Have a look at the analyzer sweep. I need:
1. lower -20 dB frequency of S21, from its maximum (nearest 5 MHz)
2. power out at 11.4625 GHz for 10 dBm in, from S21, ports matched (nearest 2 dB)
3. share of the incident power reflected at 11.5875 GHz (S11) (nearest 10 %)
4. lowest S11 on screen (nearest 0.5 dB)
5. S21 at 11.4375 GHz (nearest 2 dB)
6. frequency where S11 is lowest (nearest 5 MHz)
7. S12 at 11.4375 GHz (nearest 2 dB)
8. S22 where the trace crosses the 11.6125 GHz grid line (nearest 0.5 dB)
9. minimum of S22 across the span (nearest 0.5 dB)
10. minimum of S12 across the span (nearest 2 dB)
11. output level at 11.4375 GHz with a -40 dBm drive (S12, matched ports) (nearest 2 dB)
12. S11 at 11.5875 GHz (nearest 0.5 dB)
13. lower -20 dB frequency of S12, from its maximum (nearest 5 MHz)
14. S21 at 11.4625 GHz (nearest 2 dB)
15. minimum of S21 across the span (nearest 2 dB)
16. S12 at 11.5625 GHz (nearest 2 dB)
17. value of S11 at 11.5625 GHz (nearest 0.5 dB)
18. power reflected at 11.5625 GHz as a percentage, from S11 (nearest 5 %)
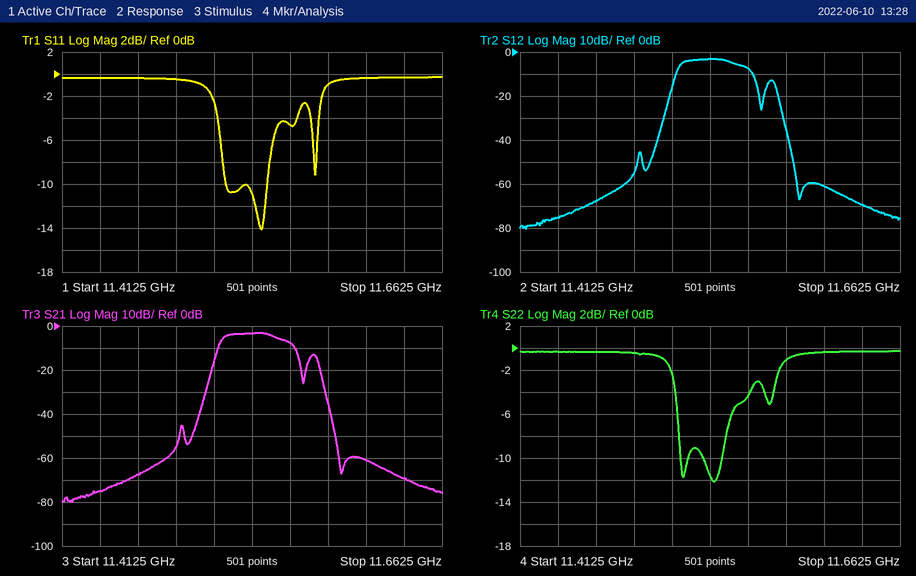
11.510 GHz
-58 dBm
80 %
-14.0 dB
-74 dB
11.545 GHz
-76 dB
-0.5 dB
-12.0 dB
-80 dB
-116 dBm
-1.0 dB
11.510 GHz
-68 dB
-80 dB
-8 dB
-4.5 dB
35 %
